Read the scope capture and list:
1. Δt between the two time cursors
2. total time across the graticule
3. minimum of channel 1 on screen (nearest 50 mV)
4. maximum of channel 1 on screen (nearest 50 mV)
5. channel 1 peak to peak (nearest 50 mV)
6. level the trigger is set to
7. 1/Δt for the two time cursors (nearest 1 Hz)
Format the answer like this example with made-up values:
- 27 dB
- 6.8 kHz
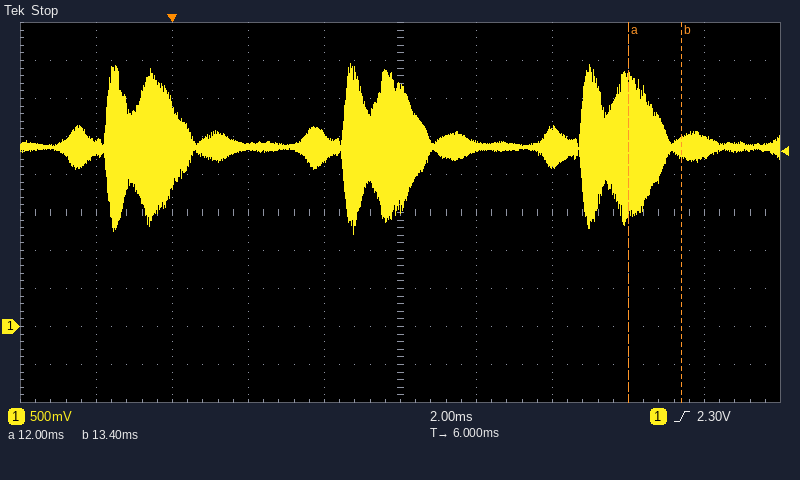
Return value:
- 1.4 ms
- 20 ms
- 1.20 V
- 3.45 V
- 2.25 V
- 2.30 V
- 714 Hz
